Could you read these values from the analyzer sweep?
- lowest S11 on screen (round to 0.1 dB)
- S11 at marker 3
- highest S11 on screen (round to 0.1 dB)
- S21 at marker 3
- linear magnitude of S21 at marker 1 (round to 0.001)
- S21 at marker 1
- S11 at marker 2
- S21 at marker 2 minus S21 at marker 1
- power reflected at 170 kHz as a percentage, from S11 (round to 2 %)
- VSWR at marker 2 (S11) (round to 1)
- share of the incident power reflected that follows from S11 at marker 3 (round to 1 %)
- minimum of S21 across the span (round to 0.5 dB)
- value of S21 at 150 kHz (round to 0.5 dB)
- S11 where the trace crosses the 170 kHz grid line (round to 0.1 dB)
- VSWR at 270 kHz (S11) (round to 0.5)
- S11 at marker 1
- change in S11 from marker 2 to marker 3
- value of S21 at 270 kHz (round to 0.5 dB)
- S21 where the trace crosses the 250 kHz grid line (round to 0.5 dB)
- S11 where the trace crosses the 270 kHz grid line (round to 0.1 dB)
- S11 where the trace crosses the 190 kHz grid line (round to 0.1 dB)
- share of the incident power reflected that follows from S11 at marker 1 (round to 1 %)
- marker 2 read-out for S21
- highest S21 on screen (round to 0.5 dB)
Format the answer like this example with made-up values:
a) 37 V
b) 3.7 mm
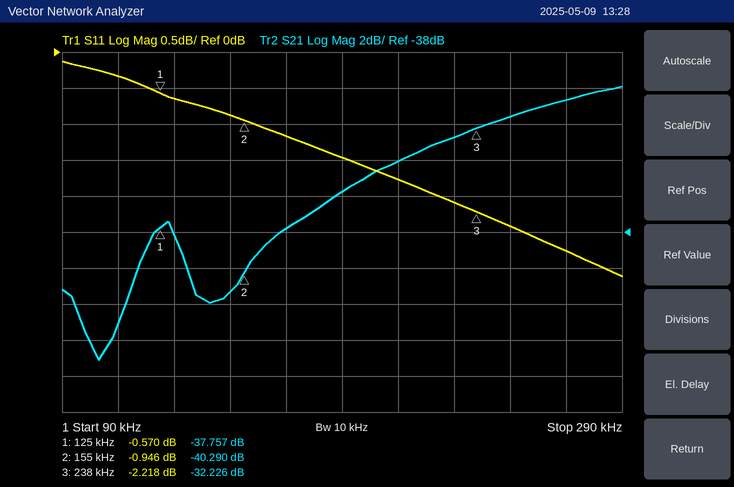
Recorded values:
a) -3.1 dB
b) -2.218 dB
c) -0.1 dB
d) -32.226 dB
e) 0.013
f) -37.757 dB
g) -0.946 dB
h) -2.533 dB
i) 76 %
j) 18
k) 60 %
l) -45.0 dB
m) -41.5 dB
n) -1.2 dB
o) 6.5
p) -0.570 dB
q) -1.272 dB
r) -30.5 dB
s) -31.5 dB
t) -2.8 dB
u) -1.5 dB
v) 88 %
w) -40.290 dB
x) -30.0 dB
